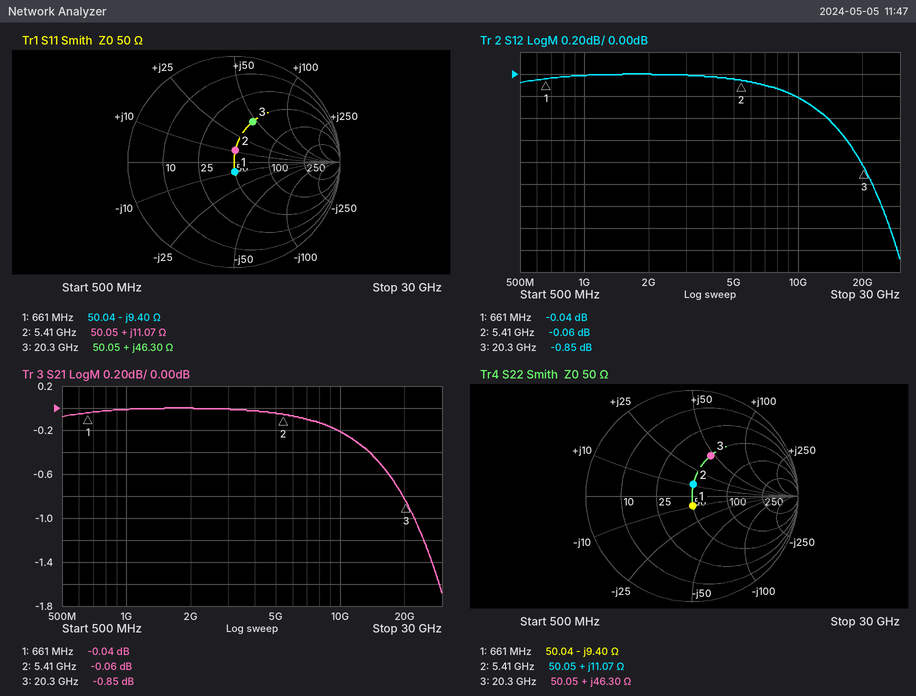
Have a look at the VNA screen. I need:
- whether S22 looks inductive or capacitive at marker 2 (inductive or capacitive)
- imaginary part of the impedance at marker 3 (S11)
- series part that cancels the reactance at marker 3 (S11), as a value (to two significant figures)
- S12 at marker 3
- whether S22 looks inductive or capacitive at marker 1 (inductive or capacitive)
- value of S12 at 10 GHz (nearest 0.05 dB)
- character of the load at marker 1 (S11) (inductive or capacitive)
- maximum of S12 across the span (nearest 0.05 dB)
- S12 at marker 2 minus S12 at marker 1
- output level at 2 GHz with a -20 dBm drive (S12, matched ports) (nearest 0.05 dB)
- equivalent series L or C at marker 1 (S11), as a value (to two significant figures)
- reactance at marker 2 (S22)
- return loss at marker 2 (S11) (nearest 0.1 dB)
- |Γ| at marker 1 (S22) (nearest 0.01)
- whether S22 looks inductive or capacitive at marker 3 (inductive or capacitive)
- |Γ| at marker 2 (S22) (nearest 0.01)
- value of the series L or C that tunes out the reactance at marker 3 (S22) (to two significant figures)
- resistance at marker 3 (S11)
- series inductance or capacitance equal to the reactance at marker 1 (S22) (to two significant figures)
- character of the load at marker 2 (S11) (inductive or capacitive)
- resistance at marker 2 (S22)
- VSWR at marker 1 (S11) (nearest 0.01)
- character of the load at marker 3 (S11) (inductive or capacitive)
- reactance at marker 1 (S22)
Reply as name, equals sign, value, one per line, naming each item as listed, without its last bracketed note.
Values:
whether S22 looks inductive or capacitive at marker 2 = inductive
imaginary part of the impedance at marker 3 = +46.30 Ω
series part that cancels the reactance at marker 3 (S11), as a value = 170 fF
S12 at marker 3 = -0.85 dB
whether S22 looks inductive or capacitive at marker 1 = capacitive
value of S12 at 10 GHz = -0.20 dB
character of the load at marker 1 (S11) = capacitive
maximum of S12 across the span = 0.00 dB
S12 at marker 2 minus S12 at marker 1 = -0.02 dB
output level at 2 GHz with a -20 dBm drive (S12, matched ports) = -20.00 dBm
equivalent series L or C at marker 1 (S11), as a value = 26 pF
reactance at marker 2 = +11.07 Ω
return loss at marker 2 (S11) = 19.2 dB
|Γ| at marker 1 (S22) = 0.09
whether S22 looks inductive or capacitive at marker 3 = inductive
|Γ| at marker 2 (S22) = 0.11
value of the series L or C that tunes out the reactance at marker 3 (S22) = 170 fF
resistance at marker 3 = 50.05 Ω
series inductance or capacitance equal to the reactance at marker 1 (S22) = 26 pF
character of the load at marker 2 (S11) = inductive
resistance at marker 2 = 50.05 Ω
VSWR at marker 1 (S11) = 1.21
character of the load at marker 3 (S11) = inductive
reactance at marker 1 = -9.40 Ω
